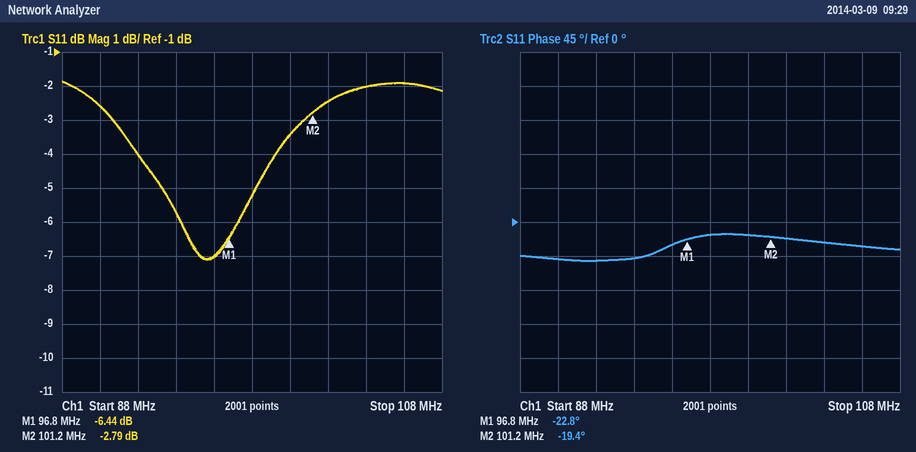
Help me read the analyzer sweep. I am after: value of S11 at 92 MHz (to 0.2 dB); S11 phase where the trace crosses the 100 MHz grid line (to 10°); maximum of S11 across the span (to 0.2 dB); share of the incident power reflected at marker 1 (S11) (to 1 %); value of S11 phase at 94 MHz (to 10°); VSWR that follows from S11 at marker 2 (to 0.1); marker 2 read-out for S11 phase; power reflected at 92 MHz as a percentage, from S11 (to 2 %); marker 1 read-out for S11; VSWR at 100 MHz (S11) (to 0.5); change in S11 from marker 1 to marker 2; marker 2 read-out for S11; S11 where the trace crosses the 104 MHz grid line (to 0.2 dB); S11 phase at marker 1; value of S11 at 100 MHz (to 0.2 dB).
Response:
-4.0 dB
-20°
-1.8 dB
23 %
-50°
6.3
-19.4°
40 %
-6.44 dB
5.0
3.65 dB
-2.79 dB
-2.0 dB
-22.8°
-3.4 dB
